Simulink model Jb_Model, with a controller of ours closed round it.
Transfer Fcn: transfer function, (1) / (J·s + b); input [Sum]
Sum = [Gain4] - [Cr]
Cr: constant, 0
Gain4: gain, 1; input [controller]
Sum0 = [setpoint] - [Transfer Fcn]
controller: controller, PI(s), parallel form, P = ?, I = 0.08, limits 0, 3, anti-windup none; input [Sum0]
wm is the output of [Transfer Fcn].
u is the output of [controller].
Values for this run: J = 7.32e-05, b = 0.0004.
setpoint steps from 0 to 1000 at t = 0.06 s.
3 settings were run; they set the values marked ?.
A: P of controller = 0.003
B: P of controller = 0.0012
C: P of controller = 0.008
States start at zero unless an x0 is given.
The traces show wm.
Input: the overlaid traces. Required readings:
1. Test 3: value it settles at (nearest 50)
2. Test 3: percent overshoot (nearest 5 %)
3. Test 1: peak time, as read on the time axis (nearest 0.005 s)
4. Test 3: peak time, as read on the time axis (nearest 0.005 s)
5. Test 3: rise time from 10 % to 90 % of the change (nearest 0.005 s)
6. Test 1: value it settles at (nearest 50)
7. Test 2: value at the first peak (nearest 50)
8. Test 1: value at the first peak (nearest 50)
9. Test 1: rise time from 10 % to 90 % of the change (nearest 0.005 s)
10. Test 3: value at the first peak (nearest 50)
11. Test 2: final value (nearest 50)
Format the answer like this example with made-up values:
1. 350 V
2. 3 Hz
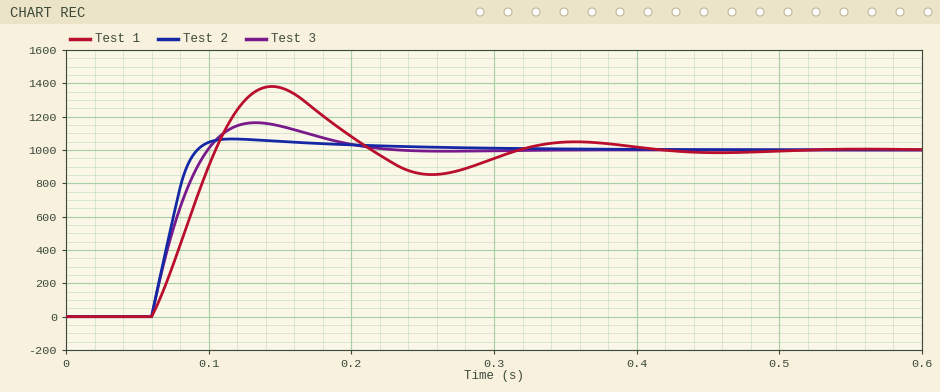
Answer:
1. 1000
2. 15 %
3. 0.145 s
4. 0.135 s
5. 0.030 s
6. 1000
7. 1050
8. 1400
9. 0.035 s
10. 1150
11. 1000
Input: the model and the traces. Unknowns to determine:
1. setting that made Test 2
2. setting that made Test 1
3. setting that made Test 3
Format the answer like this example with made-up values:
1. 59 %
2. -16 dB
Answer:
1. C
2. B
3. A
